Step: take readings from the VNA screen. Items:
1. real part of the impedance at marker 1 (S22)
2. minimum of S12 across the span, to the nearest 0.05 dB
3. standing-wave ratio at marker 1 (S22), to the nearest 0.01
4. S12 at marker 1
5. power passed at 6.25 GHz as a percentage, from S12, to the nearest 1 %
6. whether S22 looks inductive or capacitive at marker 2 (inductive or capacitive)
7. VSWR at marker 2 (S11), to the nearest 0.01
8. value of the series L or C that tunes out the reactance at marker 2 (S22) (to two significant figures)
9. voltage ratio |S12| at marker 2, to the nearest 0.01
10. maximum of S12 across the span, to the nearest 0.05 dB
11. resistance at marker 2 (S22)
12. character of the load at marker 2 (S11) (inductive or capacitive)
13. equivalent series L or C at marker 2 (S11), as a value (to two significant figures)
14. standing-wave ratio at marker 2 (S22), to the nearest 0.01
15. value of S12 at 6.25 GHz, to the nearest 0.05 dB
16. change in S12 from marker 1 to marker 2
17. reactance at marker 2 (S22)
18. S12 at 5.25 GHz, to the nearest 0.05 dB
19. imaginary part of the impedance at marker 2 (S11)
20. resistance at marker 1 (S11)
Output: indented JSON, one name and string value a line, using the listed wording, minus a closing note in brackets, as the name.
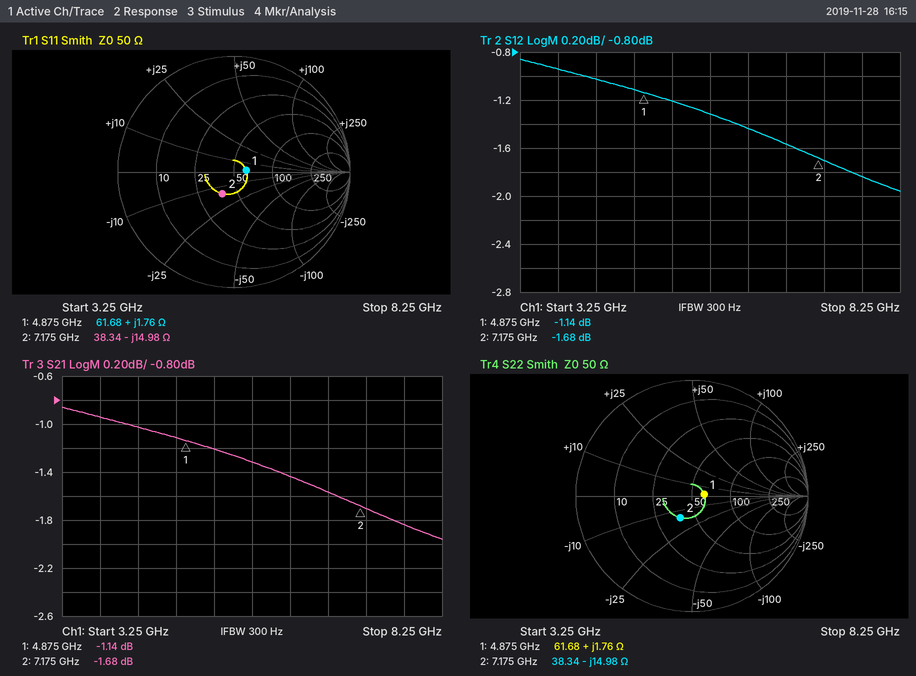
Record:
{
  "real part of the impedance at marker 1": "61.68 Ω",
  "minimum of S12 across the span, to the nearest 0.05 dB": "-1.95 dB",
  "standing-wave ratio at marker 1 (S22), to the nearest 0.01": "1.24",
  "S12 at marker 1": "-1.14 dB",
  "power passed at 6.25 GHz as a percentage, from S12, to the nearest 1 %": "72 %",
  "whether S22 looks inductive or capacitive at marker 2": "capacitive",
  "VSWR at marker 2 (S11), to the nearest 0.01": "1.54",
  "value of the series L or C that tunes out the reactance at marker 2 (S22)": "330 pH",
  "voltage ratio |S12| at marker 2, to the nearest 0.01": "0.82",
  "maximum of S12 across the span, to the nearest 0.05 dB": "-0.85 dB",
  "resistance at marker 2": "38.34 Ω",
  "character of the load at marker 2 (S11)": "capacitive",
  "equivalent series L or C at marker 2 (S11), as a value": "1.5 pF",
  "standing-wave ratio at marker 2 (S22), to the nearest 0.01": "1.54",
  "value of S12 at 6.25 GHz, to the nearest 0.05 dB": "-1.45 dB",
  "change in S12 from marker 1 to marker 2": "-0.54 dB",
  "reactance at marker 2": "-14.98 Ω",
  "S12 at 5.25 GHz, to the nearest 0.05 dB": "-1.20 dB",
  "imaginary part of the impedance at marker 2": "-14.98 Ω",
  "resistance at marker 1": "61.68 Ω"
}
